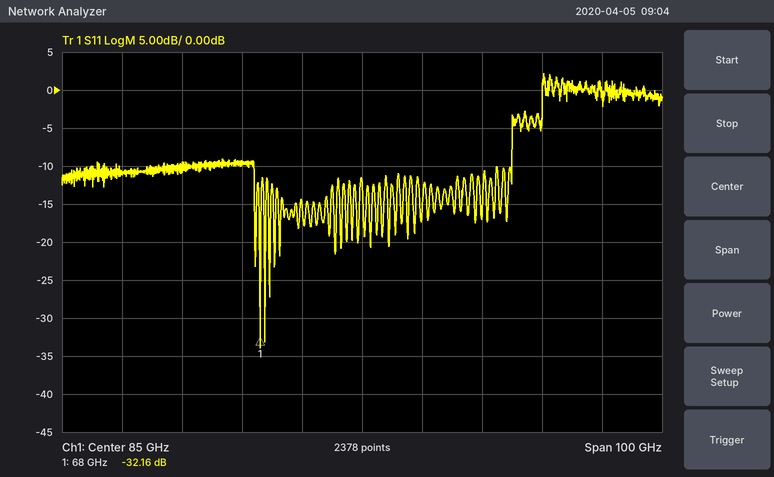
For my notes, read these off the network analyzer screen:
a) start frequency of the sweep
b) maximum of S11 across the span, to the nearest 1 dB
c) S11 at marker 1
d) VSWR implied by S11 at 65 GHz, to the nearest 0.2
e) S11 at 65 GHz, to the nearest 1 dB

35 GHz
2 dB
-32.16 dB
2.0
-10 dB
